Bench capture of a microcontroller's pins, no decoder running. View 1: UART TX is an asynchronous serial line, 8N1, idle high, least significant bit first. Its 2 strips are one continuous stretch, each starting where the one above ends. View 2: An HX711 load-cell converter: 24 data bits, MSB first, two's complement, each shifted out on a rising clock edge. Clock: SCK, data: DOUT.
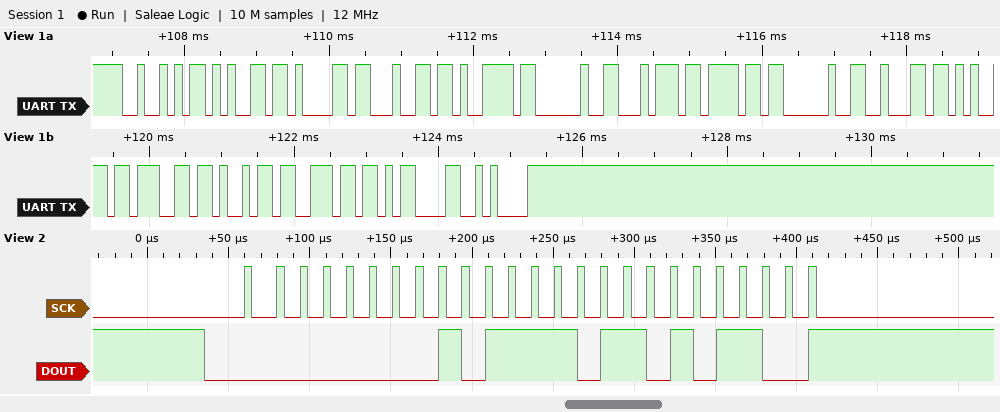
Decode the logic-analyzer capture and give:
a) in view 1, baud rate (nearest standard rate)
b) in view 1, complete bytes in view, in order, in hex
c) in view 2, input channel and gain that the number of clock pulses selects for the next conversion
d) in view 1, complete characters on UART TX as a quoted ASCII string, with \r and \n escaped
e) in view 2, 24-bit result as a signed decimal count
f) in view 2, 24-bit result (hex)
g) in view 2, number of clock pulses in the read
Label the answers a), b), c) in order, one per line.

a) 9600 baud
b) 52 65 61 64 79 20 74 6F 20 62 65 67 69 6E 0D 0A
c) channel A, gain 128
d) "Ready to begin\r\n"
e) 48556
f) 0x00BDAC
g) 25
